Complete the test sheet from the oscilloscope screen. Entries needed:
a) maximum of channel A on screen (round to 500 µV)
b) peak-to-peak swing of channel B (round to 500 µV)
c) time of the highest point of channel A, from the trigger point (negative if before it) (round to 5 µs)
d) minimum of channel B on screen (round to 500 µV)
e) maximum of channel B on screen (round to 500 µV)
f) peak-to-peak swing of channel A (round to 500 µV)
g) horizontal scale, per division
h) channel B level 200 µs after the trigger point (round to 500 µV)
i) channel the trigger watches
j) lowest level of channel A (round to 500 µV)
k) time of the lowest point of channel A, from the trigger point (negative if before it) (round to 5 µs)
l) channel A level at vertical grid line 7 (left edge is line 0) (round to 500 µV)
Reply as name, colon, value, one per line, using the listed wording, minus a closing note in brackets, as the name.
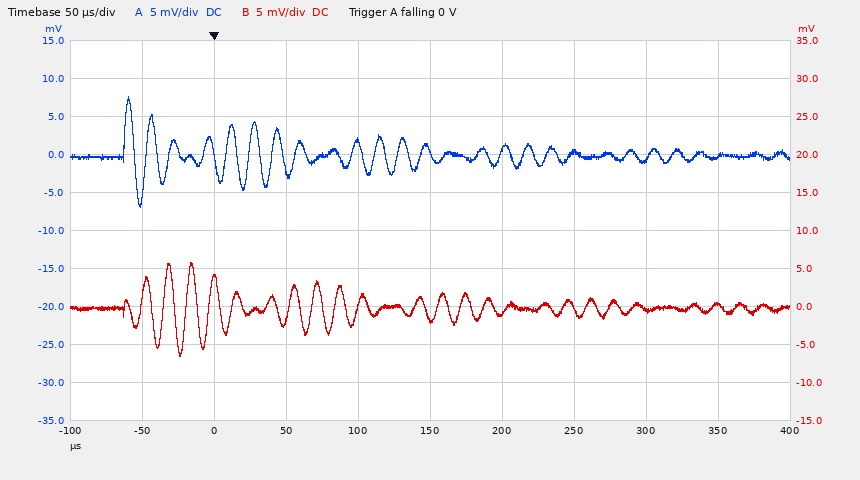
maximum of channel A on screen: 7.5 mV
peak-to-peak swing of channel B: 12.5 mV
time of the highest point of channel A, from the trigger point (negative if before it): -60 µs
minimum of channel B on screen: -6.5 mV
maximum of channel B on screen: 6.0 mV
peak-to-peak swing of channel A: 14.5 mV
horizontal scale, per division: 50 µs
channel B level 200 µs after the trigger point: -1.0 mV
channel the trigger watches: channel A
lowest level of channel A: -7.0 mV
time of the lowest point of channel A, from the trigger point (negative if before it): -50 µs
channel A level at vertical grid line 7 (left edge is line 0): 500 µV
